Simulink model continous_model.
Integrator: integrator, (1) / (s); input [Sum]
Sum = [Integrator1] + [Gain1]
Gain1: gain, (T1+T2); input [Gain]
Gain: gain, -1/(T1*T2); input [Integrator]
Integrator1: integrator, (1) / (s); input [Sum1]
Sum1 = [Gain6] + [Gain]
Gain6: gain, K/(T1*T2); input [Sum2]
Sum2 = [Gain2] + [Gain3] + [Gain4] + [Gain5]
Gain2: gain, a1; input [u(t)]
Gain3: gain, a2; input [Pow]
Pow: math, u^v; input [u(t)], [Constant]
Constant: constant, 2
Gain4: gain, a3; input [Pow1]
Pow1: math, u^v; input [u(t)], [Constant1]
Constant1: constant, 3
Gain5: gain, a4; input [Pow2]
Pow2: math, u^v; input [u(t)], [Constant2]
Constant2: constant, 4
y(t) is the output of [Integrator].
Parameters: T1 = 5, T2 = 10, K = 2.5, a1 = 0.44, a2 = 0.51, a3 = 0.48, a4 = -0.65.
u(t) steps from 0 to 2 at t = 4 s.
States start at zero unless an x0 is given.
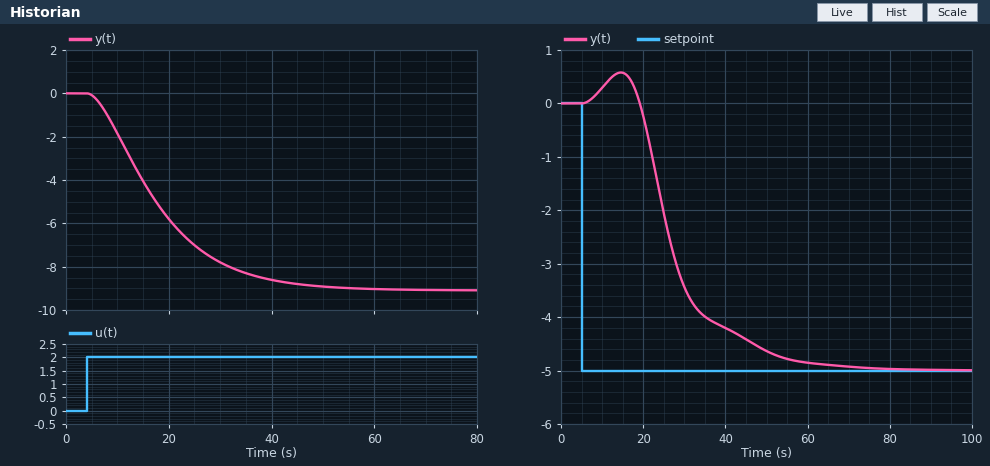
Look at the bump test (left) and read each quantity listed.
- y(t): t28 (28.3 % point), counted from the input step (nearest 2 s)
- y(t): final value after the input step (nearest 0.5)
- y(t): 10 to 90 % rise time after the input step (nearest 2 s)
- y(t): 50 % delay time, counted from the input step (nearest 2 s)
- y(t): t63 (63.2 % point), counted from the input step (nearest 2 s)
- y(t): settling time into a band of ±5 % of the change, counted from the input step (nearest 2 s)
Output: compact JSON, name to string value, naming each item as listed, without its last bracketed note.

{"y(t): t28 (28.3 % point), counted from the input step": "8 s", "y(t): final value after the input step": "-9.0", "y(t): 10 to 90 % rise time after the input step": "26 s", "y(t): 50 % delay time, counted from the input step": "12 s", "y(t): t63 (63.2 % point), counted from the input step": "16 s", "y(t): settling time into a band of ±5 % of the change, counted from the input step": "36 s"}
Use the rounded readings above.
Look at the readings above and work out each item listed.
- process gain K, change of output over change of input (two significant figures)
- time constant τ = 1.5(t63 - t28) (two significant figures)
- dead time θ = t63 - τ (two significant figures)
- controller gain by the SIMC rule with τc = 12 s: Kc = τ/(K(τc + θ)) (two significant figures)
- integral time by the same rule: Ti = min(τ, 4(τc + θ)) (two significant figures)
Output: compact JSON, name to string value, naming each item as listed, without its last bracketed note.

{"process gain K, change of output over change of input": "-4.5", "time constant τ = 1.5(t63 - t28)": "12 s", "dead time θ = t63 - τ": "4.0 s", "controller gain by the SIMC rule with τc = 12 s: Kc = τ/(K(τc + θ))": "-0.17", "integral time by the same rule: Ti = min(τ, 4(τc + θ))": "12 s"}
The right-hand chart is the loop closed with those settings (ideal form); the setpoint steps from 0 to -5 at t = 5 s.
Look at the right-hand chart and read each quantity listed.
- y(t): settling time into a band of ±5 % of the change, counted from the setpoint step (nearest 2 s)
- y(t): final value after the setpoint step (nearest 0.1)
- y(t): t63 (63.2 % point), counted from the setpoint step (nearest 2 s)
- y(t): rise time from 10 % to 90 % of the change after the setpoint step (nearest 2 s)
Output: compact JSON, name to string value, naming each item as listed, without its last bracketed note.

{"y(t): settling time into a band of ±5 % of the change, counted from the setpoint step": "48 s", "y(t): final value after the setpoint step": "-5.0", "y(t): t63 (63.2 % point), counted from the setpoint step": "24 s", "y(t): rise time from 10 % to 90 % of the change after the setpoint step": "26 s"}
